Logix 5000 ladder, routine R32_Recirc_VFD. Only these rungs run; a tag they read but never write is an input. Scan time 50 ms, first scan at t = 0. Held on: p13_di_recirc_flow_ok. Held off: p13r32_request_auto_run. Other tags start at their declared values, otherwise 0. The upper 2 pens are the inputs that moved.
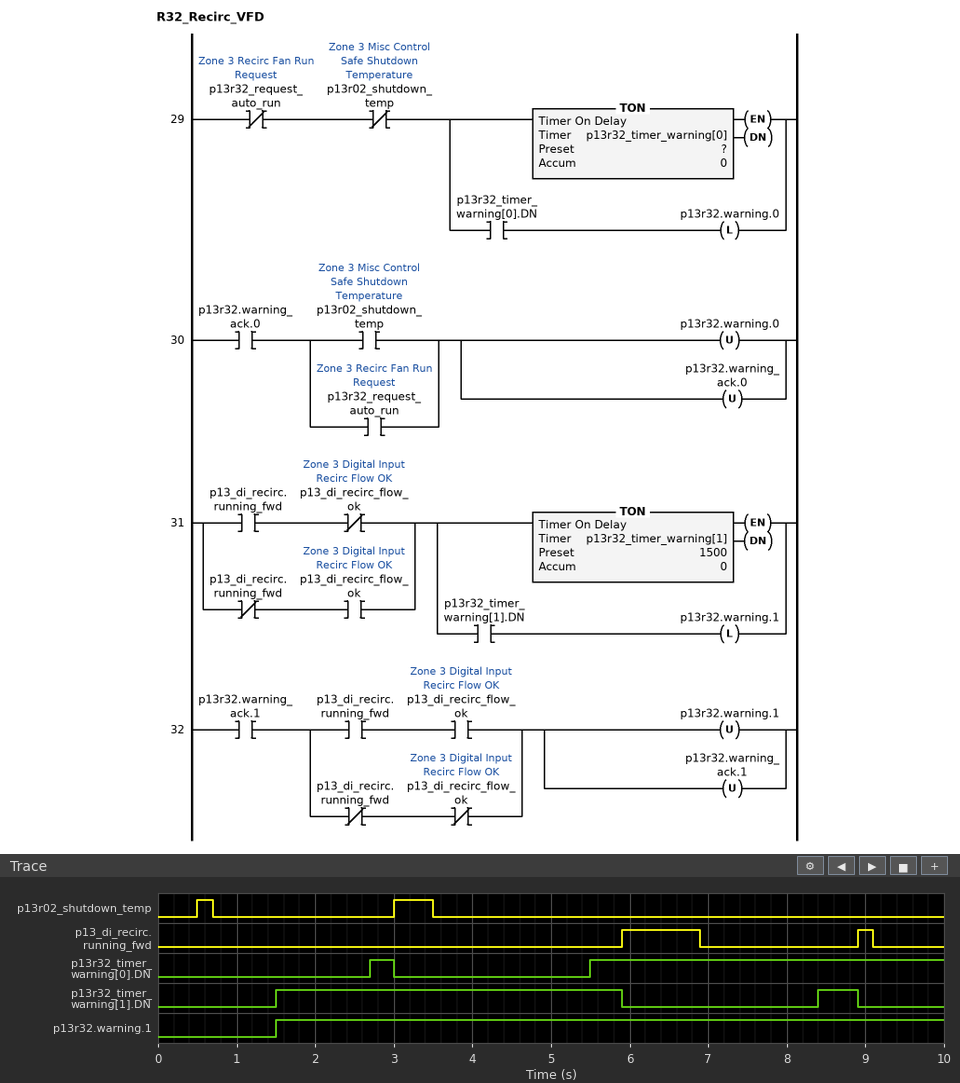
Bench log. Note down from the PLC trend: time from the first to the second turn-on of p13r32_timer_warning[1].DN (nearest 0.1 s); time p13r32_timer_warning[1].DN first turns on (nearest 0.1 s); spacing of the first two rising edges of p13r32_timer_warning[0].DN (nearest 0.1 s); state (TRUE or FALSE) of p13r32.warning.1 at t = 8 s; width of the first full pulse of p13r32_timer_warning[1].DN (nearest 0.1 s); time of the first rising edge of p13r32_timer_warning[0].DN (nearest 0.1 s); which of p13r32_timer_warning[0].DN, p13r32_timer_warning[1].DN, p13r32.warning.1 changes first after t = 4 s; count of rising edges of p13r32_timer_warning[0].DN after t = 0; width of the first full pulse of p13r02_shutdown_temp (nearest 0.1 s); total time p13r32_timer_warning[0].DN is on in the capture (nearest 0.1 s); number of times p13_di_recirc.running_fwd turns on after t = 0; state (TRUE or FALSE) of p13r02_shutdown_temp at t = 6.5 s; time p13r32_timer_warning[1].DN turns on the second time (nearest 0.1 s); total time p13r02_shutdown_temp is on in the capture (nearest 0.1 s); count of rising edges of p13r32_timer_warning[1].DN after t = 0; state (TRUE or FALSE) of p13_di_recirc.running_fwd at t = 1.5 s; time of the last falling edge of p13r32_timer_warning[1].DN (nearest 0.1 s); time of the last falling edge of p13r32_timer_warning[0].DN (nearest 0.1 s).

6.9 s
1.5 s
2.8 s
TRUE
4.4 s
2.7 s
p13r32_timer_warning[0].DN
2
0.2 s
4.8 s
2
FALSE
8.4 s
0.7 s
2
FALSE
8.9 s
3.0 s
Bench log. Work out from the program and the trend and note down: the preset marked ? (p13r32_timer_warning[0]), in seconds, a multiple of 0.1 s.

2.0 s
